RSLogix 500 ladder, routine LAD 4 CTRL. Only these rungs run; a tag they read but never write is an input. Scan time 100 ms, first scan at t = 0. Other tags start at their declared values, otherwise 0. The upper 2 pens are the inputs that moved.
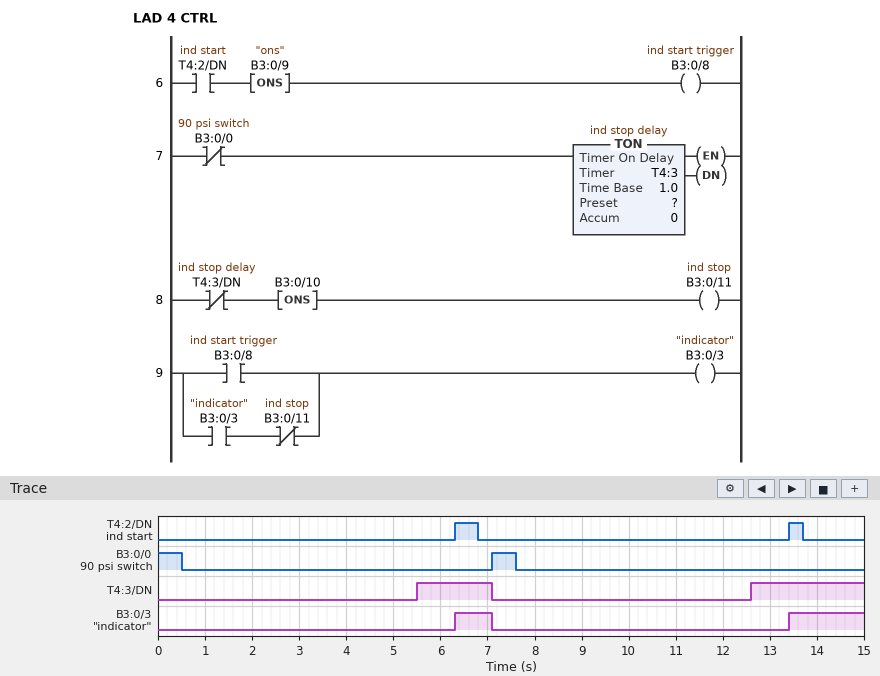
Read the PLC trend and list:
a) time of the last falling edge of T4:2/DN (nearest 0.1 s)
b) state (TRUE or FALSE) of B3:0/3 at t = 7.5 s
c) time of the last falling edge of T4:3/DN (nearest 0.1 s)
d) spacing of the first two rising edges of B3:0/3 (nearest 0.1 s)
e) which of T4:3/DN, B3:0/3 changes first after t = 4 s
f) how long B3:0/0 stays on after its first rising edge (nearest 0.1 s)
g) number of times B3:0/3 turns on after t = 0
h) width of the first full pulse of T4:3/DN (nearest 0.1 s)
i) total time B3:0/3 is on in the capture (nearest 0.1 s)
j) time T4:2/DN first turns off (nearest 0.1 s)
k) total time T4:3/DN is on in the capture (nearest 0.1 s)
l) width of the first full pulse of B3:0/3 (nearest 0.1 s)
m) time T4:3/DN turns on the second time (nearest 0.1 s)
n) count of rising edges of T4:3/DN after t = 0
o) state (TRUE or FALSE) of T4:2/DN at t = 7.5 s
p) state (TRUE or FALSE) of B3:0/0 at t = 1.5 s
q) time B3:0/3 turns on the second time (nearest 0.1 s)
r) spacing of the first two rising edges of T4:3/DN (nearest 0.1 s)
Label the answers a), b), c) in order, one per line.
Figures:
a) 13.7 s
b) FALSE
c) 7.1 s
d) 7.1 s
e) T4:3/DN
f) 0.5 s
g) 2
h) 1.6 s
i) 2.4 s
j) 6.8 s
k) 4.0 s
l) 0.8 s
m) 12.6 s
n) 2
o) FALSE
p) FALSE
q) 13.4 s
r) 7.1 s
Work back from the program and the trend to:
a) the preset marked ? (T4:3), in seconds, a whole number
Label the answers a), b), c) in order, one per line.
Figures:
a) 5 s
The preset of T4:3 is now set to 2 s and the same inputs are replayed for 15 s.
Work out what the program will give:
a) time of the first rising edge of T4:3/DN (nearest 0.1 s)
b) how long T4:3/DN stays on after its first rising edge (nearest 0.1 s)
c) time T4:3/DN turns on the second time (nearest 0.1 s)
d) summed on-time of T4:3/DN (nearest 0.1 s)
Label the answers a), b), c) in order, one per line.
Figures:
a) 2.5 s
b) 4.6 s
c) 9.6 s
d) 10.0 s
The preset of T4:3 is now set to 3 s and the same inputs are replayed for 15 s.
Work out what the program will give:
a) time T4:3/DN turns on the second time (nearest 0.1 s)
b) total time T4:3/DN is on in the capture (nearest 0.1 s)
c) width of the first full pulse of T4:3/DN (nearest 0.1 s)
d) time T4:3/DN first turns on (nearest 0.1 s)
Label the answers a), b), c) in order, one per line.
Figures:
a) 10.6 s
b) 8.0 s
c) 3.6 s
d) 3.5 s
